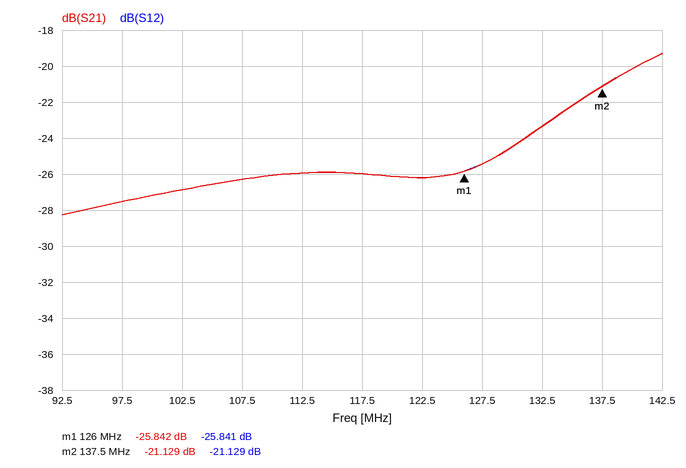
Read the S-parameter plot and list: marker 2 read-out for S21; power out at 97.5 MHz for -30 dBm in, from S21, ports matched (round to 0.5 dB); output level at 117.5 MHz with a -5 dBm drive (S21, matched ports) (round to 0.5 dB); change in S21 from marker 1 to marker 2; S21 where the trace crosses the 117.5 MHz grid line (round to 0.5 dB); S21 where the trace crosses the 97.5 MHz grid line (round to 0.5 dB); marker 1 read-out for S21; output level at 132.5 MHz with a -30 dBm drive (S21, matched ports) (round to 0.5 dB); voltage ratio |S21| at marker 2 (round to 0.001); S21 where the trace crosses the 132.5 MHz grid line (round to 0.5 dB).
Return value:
-21.129 dB
-57.5 dBm
-31.0 dBm
4.713 dB
-26.0 dB
-27.5 dB
-25.842 dB
-53.5 dBm
0.088
-23.5 dB
